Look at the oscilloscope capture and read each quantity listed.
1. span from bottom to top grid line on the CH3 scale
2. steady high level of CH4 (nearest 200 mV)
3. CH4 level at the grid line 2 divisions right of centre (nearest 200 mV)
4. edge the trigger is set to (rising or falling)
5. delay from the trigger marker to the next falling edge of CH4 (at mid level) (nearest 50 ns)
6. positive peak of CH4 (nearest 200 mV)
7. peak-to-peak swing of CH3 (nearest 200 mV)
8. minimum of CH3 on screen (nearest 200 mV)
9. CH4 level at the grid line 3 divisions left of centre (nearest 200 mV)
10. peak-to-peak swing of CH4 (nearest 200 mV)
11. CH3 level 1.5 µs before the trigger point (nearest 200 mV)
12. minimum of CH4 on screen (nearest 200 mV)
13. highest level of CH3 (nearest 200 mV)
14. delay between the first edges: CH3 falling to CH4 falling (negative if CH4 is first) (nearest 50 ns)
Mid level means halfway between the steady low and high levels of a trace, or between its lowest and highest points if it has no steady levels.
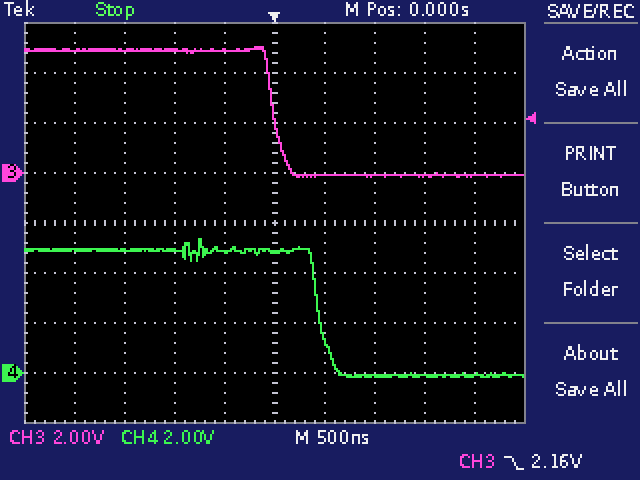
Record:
16 V
5.0 V
-200 mV
falling
450 ns
5.4 V
5.2 V
-200 mV
5.0 V
5.6 V
5.0 V
-200 mV
5.0 V
+450 ns
